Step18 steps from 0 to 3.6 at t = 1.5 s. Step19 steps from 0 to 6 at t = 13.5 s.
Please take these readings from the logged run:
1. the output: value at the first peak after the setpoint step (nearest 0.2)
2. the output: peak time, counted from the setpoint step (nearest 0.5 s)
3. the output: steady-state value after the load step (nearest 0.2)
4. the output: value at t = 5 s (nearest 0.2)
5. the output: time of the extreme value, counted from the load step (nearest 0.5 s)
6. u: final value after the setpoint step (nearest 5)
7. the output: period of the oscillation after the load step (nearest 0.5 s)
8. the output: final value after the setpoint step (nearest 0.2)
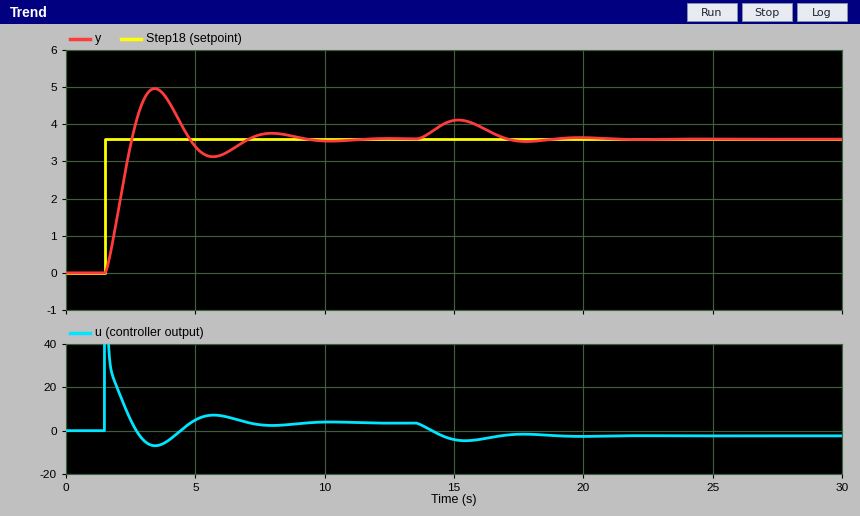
5.0
2.0 s
3.6
3.4
1.5 s
5
4.5 s
3.6
